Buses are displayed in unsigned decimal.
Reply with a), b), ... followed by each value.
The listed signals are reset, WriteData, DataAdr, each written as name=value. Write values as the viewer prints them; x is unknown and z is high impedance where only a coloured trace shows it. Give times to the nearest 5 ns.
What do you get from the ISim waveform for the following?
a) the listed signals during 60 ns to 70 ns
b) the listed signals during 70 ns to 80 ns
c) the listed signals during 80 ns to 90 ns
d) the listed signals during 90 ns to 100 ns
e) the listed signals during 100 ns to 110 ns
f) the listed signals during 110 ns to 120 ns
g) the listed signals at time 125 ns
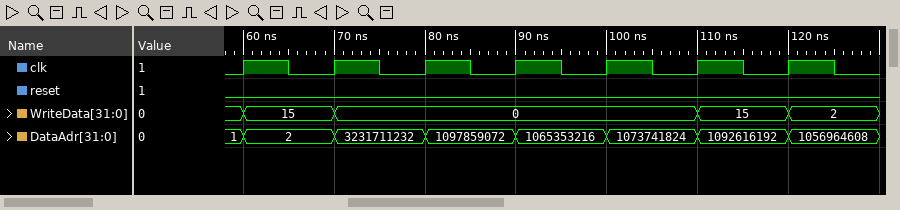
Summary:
a) reset=0, WriteData=15, DataAdr=2
b) reset=0, WriteData=0, DataAdr=3231711232
c) reset=0, WriteData=0, DataAdr=1097859072
d) reset=0, WriteData=0, DataAdr=1065353216
e) reset=0, WriteData=0, DataAdr=1073741824
f) reset=0, WriteData=15, DataAdr=1092616192
g) reset=0, WriteData=2, DataAdr=1056964608
